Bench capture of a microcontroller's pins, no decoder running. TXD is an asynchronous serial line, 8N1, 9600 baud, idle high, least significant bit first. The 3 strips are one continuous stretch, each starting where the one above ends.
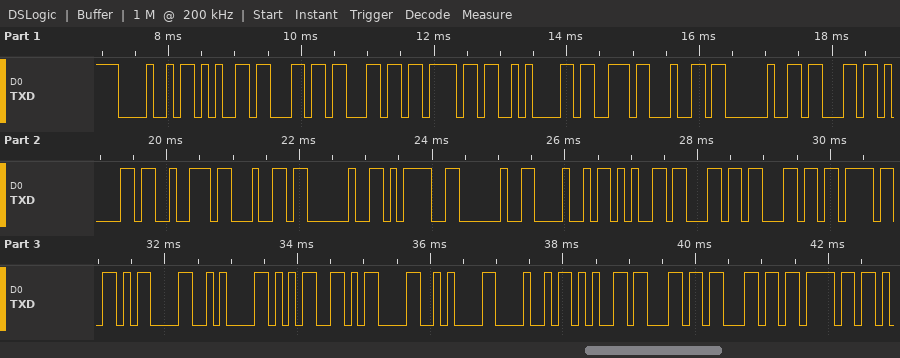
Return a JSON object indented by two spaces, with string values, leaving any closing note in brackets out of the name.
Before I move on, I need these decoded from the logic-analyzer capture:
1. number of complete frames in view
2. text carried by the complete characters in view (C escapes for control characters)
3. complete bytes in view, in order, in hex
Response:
{
  "number of complete frames in view": "31",
  "text carried by the complete characters in view": "\"Hello\\nsd card = Hello\\r\\n5\\r\\nHello\"",
  "complete bytes in view, in order, in hex": "48 65 6C 6C 6F 0A 73 64 20 63 61 72 64 20 3D 20 48 65 6C 6C 6F 0D 0A 35 0D 0A 48 65 6C 6C 6F"
}
